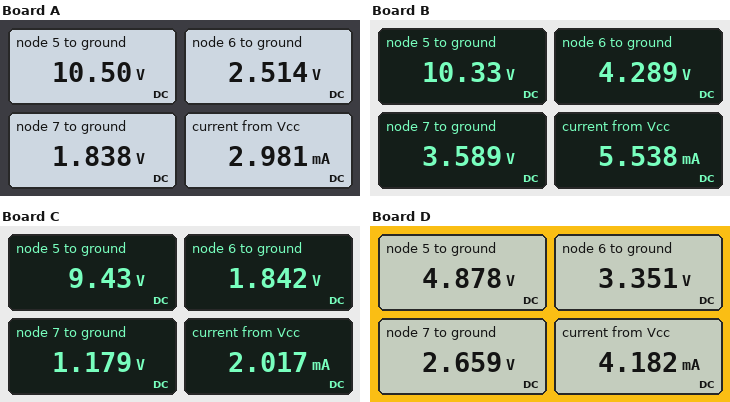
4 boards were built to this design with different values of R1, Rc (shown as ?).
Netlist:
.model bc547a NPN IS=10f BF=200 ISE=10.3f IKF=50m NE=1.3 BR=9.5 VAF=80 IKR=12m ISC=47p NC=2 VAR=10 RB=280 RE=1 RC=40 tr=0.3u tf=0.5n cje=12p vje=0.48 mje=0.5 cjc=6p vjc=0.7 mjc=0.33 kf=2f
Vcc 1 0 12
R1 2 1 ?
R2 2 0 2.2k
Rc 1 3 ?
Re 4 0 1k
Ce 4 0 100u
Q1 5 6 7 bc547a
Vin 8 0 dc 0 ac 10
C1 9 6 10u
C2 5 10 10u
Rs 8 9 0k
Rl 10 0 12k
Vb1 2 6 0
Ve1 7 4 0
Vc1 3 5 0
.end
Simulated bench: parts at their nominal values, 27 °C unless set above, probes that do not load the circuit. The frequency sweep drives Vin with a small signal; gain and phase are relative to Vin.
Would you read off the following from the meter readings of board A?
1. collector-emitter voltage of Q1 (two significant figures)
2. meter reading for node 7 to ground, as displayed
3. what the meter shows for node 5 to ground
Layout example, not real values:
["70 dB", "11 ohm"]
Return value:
["8.7 V", "1.838 V", "10.50 V"]
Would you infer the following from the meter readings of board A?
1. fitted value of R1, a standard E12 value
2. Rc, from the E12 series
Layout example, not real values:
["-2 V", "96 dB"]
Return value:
["8.2 kΩ", "820 Ω"]
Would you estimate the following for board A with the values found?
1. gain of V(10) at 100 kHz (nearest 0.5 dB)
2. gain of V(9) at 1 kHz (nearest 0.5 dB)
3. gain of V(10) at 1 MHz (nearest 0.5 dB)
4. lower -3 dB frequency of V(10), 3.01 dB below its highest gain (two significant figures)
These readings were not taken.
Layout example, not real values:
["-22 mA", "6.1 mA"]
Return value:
["32.5 dB", "0 dB", "32.0 dB", "98 Hz"]
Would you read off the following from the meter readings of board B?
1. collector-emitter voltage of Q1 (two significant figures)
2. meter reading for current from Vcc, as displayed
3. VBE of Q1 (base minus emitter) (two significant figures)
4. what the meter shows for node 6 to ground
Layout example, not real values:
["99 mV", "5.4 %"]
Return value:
["6.7 V", "5.538 mA", "700 mV", "4.289 V"]
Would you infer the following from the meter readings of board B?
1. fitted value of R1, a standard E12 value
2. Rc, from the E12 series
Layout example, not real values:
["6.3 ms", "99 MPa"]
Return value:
["3.9 kΩ", "470 Ω"]
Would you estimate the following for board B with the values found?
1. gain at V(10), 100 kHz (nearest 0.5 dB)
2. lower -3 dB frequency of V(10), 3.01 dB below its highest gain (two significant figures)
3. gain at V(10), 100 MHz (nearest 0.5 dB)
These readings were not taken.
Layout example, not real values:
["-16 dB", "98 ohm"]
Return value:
["32.0 dB", "160 Hz", "1.0 dB"]
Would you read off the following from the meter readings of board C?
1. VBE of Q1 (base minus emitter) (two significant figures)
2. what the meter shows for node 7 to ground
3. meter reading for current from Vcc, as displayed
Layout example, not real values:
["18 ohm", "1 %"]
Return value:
["660 mV", "1.179 V", "2.017 mA"]
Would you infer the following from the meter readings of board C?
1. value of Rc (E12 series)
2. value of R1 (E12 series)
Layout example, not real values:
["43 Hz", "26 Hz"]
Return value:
["2.2 kΩ", "12 kΩ"]
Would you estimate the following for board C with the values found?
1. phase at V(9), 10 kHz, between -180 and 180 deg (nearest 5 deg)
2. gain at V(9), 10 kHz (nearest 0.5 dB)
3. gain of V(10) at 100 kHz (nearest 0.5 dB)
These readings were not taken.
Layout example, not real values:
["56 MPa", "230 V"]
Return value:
["0 deg", "0 dB", "37.0 dB"]
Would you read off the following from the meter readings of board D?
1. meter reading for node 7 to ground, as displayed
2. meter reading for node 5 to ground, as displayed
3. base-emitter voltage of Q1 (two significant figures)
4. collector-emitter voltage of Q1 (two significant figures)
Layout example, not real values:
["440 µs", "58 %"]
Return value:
["2.659 V", "4.878 V", "690 mV", "2.2 V"]
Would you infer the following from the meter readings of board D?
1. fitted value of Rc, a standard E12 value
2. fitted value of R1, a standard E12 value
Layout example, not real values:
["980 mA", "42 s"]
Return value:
["2.7 kΩ", "5.6 kΩ"]
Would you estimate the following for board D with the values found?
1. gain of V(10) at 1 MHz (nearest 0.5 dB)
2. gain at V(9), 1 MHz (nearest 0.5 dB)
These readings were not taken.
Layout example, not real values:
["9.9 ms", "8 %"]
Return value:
["39.5 dB", "0 dB"]
